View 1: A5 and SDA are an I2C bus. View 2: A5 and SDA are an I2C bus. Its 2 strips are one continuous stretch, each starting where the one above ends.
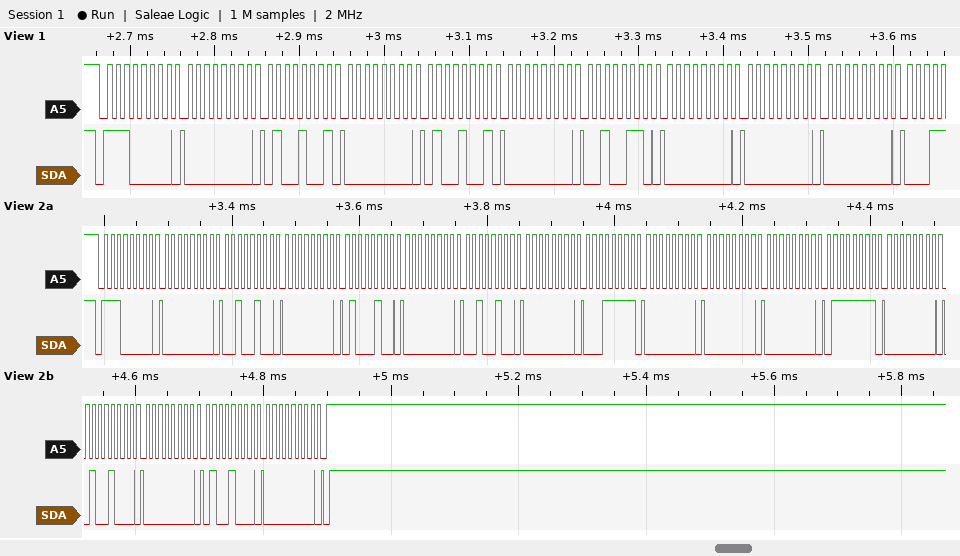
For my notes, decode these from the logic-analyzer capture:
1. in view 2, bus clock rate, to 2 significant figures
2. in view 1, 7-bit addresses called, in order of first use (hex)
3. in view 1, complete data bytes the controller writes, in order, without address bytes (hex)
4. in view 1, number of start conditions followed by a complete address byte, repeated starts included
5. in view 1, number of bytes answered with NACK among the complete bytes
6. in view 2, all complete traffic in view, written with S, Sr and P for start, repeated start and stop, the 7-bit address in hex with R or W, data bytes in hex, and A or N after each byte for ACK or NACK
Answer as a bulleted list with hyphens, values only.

- 100 kHz
- 0x70
- 00 49 00 49 00 26 00 00 00
- 1
- 0
- S 70W A 00 A 24 A 00 A 44 A 00 A 24 A 00 A 1F A 00 A 00 A 00 A 7F A 00 A 48 A 00 A 48 A 00 A P
